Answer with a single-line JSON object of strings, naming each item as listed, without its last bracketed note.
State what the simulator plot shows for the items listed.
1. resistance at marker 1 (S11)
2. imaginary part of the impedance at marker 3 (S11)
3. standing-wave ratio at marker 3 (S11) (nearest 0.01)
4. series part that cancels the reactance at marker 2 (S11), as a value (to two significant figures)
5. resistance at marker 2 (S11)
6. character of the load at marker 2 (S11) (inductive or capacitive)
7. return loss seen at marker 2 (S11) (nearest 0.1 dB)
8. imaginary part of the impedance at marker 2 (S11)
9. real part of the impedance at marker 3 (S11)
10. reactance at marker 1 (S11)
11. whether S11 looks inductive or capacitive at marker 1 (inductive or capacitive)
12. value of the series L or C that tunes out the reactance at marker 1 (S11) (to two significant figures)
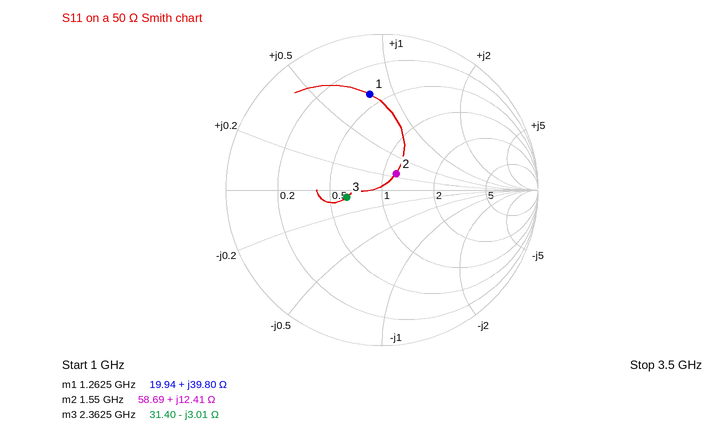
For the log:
{"resistance at marker 1": "19.94 Ω", "imaginary part of the impedance at marker 3": "-3.01 Ω", "standing-wave ratio at marker 3 (S11)": "1.60", "series part that cancels the reactance at marker 2 (S11), as a value": "8.3 pF", "resistance at marker 2": "58.69 Ω", "character of the load at marker 2 (S11)": "inductive", "return loss seen at marker 2 (S11)": "17.2 dB", "imaginary part of the impedance at marker 2": "+12.41 Ω", "real part of the impedance at marker 3": "31.40 Ω", "reactance at marker 1": "+39.80 Ω", "whether S11 looks inductive or capacitive at marker 1": "inductive", "value of the series L or C that tunes out the reactance at marker 1 (S11)": "3.2 pF"}
